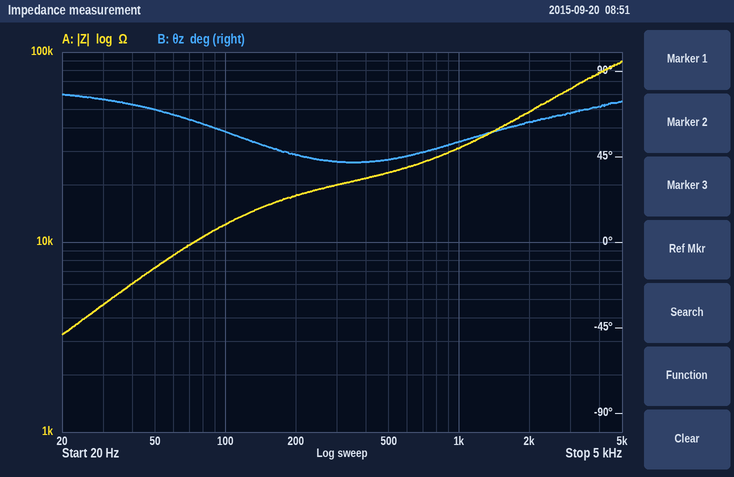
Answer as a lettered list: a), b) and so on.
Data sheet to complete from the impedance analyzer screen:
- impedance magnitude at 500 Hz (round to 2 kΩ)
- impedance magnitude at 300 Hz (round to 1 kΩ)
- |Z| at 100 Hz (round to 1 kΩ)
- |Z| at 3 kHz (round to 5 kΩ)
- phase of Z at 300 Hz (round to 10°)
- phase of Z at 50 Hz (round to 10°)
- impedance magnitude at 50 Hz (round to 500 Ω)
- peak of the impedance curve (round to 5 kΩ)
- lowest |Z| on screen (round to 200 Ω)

a) 24 kΩ
b) 20 kΩ
c) 12 kΩ
d) 65 kΩ
e) 40°
f) 70°
g) 7.5 kΩ
h) 90 kΩ
i) 3.2 kΩ
